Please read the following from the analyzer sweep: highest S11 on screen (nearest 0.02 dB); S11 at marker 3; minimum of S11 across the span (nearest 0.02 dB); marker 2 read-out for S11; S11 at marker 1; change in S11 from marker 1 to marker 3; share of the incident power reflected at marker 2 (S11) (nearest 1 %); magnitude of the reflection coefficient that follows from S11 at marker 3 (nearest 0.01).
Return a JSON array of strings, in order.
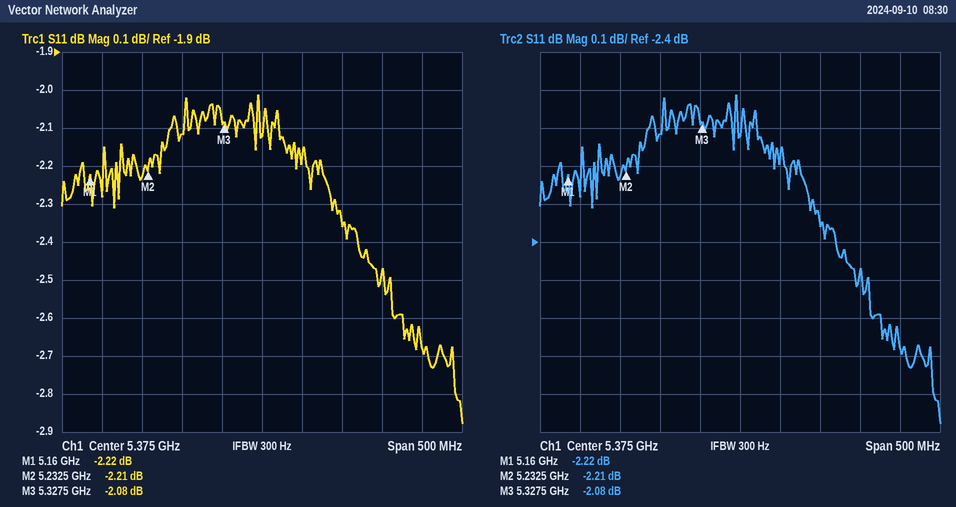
["-2.02 dB", "-2.08 dB", "-2.88 dB", "-2.21 dB", "-2.22 dB", "0.14 dB", "60 %", "0.79"]
